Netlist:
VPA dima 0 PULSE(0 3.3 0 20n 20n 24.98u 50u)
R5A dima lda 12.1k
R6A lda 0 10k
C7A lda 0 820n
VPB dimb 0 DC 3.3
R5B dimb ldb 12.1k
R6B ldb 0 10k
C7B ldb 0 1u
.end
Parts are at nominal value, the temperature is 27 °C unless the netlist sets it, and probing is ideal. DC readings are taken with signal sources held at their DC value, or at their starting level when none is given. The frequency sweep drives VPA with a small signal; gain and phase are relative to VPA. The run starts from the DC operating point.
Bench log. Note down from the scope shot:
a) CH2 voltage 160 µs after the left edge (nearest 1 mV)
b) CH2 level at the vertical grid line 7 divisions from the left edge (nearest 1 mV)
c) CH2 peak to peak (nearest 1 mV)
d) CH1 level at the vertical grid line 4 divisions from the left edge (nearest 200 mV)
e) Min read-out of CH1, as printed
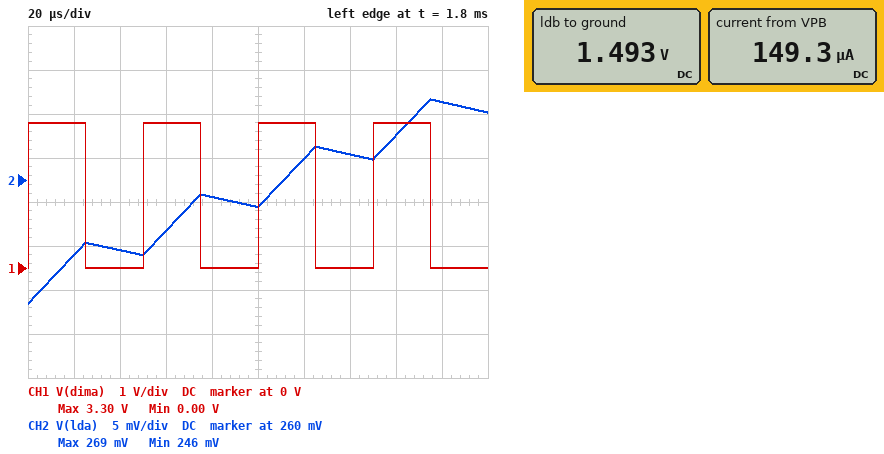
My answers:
265 mV
263 mV
23 mV
0 V
0.00 V
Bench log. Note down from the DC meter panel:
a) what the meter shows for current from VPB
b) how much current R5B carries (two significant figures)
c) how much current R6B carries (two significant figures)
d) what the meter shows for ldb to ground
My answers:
149.3 µA
150 µA
150 µA
1.493 V
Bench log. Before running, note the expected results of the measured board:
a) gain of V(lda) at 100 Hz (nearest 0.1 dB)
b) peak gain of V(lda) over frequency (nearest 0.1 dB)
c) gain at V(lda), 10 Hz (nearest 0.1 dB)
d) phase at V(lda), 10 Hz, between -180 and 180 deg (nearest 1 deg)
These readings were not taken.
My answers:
-16.4 dB
-6.9 dB
-7.2 dB
-16 deg
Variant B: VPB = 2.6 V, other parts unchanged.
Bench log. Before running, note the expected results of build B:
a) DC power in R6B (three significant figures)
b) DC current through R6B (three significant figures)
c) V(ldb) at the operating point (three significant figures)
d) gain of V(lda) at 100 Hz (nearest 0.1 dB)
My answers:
138 µW
118 µA
1.18 V
-16.4 dB
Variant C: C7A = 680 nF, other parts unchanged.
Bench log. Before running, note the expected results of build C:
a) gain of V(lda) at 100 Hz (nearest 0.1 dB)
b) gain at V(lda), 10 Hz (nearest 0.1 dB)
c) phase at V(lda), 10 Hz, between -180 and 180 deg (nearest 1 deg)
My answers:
-15.0 dB
-7.1 dB
-13 deg
